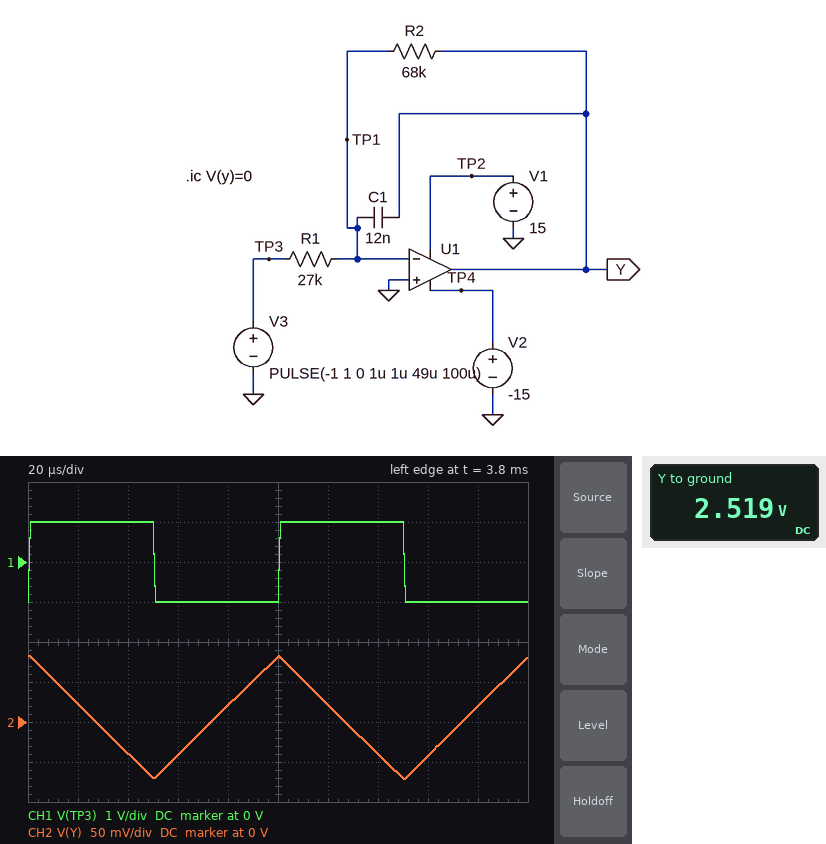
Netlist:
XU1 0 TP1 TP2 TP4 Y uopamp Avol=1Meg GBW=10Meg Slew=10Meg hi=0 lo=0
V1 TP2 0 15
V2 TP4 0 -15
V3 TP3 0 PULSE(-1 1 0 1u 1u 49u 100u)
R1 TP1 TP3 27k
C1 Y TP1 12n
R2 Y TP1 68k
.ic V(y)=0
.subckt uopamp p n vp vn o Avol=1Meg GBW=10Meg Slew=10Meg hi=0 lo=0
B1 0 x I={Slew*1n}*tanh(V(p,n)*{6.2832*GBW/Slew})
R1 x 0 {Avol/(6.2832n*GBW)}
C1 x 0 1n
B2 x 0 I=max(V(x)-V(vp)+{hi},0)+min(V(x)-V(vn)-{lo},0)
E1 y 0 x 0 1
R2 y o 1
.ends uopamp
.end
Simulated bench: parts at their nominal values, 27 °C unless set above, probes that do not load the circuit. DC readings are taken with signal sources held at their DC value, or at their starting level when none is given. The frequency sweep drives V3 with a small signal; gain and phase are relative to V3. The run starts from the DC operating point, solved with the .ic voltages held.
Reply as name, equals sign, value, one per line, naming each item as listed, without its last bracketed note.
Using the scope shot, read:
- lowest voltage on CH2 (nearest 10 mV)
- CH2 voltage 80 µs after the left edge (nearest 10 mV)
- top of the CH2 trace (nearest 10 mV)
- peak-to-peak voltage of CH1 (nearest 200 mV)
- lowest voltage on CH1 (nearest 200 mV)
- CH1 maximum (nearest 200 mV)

lowest voltage on CH2 = -70 mV
CH2 voltage 80 µs after the left edge = 20 mV
top of the CH2 trace = 80 mV
peak-to-peak voltage of CH1 = 2.0 V
lowest voltage on CH1 = -1.0 V
CH1 maximum = 1.0 V
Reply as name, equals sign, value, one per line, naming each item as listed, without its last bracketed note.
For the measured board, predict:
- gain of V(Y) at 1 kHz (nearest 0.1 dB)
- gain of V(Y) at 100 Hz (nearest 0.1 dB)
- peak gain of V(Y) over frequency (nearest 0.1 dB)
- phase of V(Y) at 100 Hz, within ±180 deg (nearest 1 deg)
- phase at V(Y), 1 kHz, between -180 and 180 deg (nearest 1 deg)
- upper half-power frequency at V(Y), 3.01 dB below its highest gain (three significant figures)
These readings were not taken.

gain of V(Y) at 1 kHz = -6.3 dB
gain of V(Y) at 100 Hz = 7.0 dB
peak gain of V(Y) over frequency = 8.0 dB
phase of V(Y) at 100 Hz, within ±180 deg = 153 deg
phase at V(Y), 1 kHz, between -180 and 180 deg = 101 deg
upper half-power frequency at V(Y), 3.01 dB below its highest gain = 195 Hz
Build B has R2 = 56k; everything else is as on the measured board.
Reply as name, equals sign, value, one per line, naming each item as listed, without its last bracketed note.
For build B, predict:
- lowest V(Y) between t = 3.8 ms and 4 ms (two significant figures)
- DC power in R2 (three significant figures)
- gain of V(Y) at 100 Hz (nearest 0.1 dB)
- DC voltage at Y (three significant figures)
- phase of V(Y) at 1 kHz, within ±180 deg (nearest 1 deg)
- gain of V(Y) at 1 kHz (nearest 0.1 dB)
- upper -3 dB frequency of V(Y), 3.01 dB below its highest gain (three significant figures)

lowest V(Y) between t = 3.8 ms and 4 ms = -75 mV
DC power in R2 = 76.8 µW
gain of V(Y) at 100 Hz = 5.6 dB
DC voltage at Y = 2.07 V
phase of V(Y) at 1 kHz, within ±180 deg = 103 deg
gain of V(Y) at 1 kHz = -6.4 dB
upper -3 dB frequency of V(Y), 3.01 dB below its highest gain = 237 Hz
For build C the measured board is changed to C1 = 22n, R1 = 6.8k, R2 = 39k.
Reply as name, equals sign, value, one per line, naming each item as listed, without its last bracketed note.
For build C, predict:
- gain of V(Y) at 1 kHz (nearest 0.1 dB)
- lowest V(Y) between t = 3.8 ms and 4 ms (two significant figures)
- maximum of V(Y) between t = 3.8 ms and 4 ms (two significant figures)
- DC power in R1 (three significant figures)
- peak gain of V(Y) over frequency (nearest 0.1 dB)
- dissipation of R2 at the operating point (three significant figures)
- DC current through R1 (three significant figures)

gain of V(Y) at 1 kHz = 0.4 dB
lowest V(Y) between t = 3.8 ms and 4 ms = -160 mV
maximum of V(Y) between t = 3.8 ms and 4 ms = 170 mV
DC power in R1 = 147 µW
peak gain of V(Y) over frequency = 15.2 dB
dissipation of R2 at the operating point = 843 µW
DC current through R1 = 147 µA
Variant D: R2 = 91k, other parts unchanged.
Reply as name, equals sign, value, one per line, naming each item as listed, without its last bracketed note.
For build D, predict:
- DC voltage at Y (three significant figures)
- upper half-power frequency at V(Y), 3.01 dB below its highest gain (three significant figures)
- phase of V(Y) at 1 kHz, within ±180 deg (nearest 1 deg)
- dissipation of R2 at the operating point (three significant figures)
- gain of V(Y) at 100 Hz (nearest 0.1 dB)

DC voltage at Y = 3.37 V
upper half-power frequency at V(Y), 3.01 dB below its highest gain = 146 Hz
phase of V(Y) at 1 kHz, within ±180 deg = 98 deg
dissipation of R2 at the operating point = 125 µW
gain of V(Y) at 100 Hz = 8.9 dB
